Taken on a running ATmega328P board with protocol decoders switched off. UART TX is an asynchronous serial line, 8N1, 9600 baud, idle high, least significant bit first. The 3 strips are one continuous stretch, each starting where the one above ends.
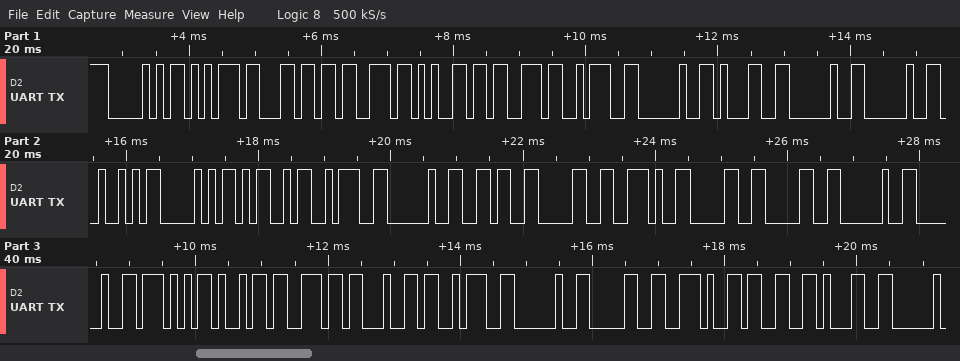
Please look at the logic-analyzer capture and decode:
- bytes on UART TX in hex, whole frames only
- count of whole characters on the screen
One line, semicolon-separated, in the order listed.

0x50 0x75 0x6C 0x73 0x65 0x73 0x3A 0x20 0x31 0x20 0x20 0x52 0x50 0x4D 0x3A 0x20 0x36 0x30 0x2E 0x30 0x30 0x20 0x20 0x57 0x69 0x6E 0x64 0x3A 0x20 0x30 0x2E 0x33 0x31; 33
